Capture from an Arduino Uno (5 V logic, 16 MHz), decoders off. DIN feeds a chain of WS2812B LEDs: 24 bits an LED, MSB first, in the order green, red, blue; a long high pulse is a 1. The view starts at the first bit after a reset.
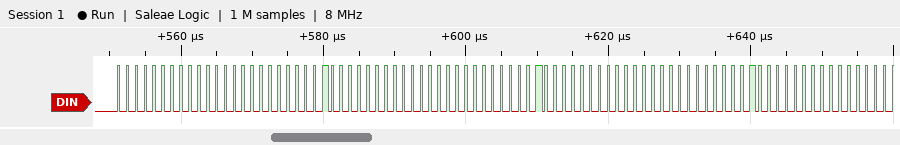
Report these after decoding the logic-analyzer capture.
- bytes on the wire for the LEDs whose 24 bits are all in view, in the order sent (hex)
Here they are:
00 00 01 00 00 01 00 00 01
